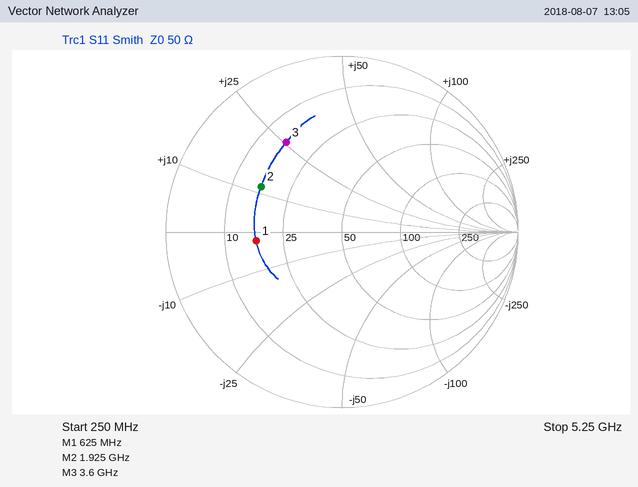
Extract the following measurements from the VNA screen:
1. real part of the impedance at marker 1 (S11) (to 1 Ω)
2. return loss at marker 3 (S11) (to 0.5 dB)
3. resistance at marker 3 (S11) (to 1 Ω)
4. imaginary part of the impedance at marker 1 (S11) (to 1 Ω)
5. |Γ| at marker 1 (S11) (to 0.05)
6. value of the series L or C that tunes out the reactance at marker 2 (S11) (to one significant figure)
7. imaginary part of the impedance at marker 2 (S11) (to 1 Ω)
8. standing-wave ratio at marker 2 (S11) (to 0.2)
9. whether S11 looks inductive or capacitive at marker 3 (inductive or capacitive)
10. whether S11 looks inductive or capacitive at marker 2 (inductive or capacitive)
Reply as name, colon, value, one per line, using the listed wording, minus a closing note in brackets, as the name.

real part of the impedance at marker 1 (S11): 17 Ω
return loss at marker 3 (S11): 4.5 dB
resistance at marker 3 (S11): 16 Ω
imaginary part of the impedance at marker 1 (S11): -2 Ω
|Γ| at marker 1 (S11): 0.50
value of the series L or C that tunes out the reactance at marker 2 (S11): 7 pF
imaginary part of the impedance at marker 2 (S11): +12 Ω
standing-wave ratio at marker 2 (S11): 3.2
whether S11 looks inductive or capacitive at marker 3: inductive
whether S11 looks inductive or capacitive at marker 2: inductive
